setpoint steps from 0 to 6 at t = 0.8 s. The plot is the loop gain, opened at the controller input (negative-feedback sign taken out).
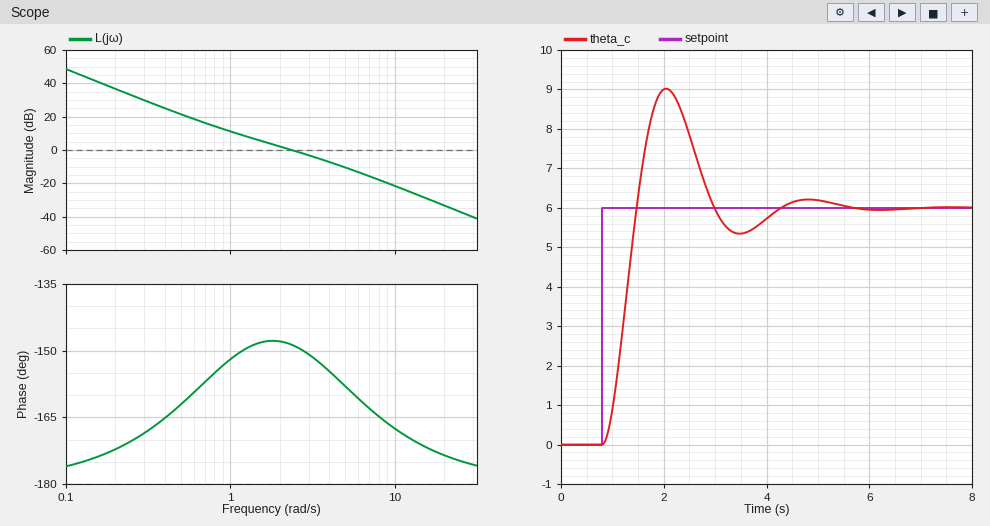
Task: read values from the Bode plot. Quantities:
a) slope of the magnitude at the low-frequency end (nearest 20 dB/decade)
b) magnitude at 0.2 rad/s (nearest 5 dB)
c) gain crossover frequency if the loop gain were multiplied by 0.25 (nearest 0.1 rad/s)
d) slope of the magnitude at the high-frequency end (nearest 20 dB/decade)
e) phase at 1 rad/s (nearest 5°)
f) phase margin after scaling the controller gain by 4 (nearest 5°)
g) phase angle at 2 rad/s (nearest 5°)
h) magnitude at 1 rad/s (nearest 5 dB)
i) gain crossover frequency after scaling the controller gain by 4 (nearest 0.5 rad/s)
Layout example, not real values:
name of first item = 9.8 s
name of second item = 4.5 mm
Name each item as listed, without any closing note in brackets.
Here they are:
slope of the magnitude at the low-frequency end = -40 dB/decade
magnitude at 0.2 rad/s = 35 dB
gain crossover frequency if the loop gain were multiplied by 0.25 = 0.9 rad/s
slope of the magnitude at the high-frequency end = -40 dB/decade
phase at 1 rad/s = -150°
phase margin after scaling the controller gain by 4 = 20°
phase angle at 2 rad/s = -150°
magnitude at 1 rad/s = 10 dB
gain crossover frequency after scaling the controller gain by 4 = 5.5 rad/s
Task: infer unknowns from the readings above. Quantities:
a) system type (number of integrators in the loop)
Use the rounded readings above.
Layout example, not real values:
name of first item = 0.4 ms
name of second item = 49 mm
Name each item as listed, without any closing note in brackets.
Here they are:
system type = 2
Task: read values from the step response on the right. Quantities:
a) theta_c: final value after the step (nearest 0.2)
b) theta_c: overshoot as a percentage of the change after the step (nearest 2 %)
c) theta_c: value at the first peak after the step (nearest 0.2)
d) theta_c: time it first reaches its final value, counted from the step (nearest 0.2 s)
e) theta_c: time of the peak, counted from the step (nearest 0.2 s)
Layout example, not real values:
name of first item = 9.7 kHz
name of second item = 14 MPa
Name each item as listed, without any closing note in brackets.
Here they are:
theta_c: final value after the step = 6.0
theta_c: overshoot as a percentage of the change after the step = 50 %
theta_c: value at the first peak after the step = 9.0
theta_c: time it first reaches its final value, counted from the step = 0.6 s
theta_c: time of the peak, counted from the step = 1.2 s
